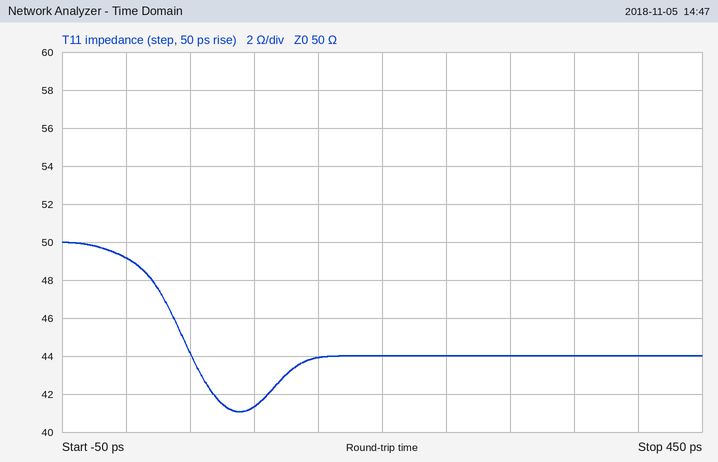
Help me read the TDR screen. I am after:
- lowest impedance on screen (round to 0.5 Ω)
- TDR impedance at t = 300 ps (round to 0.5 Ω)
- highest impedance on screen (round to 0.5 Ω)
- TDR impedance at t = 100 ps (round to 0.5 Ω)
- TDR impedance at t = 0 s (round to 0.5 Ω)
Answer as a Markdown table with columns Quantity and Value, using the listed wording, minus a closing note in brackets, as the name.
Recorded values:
| Quantity | Value |
|---|---|
| lowest impedance on screen | 41.0 Ω |
| TDR impedance at t = 300 ps | 44.0 Ω |
| highest impedance on screen | 50.0 Ω |
| TDR impedance at t = 100 ps | 41.5 Ω |
| TDR impedance at t = 0 s | 49.0 Ω |
